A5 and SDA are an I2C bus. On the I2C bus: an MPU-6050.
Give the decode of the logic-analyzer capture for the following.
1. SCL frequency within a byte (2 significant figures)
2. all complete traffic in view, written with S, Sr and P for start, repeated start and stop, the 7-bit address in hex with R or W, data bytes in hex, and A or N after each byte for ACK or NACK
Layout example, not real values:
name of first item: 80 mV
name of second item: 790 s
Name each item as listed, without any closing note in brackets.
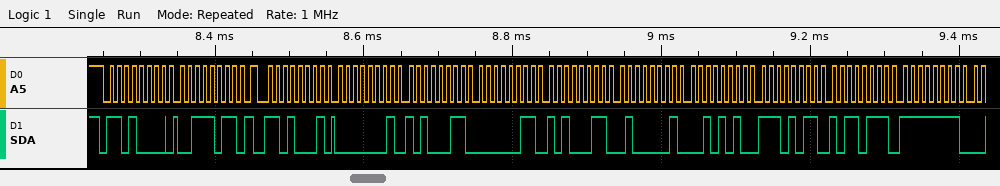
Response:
SCL frequency within a byte: 100 kHz
all complete traffic in view, written with S, Sr and P for start, repeated start and stop, the 7-bit address in hex with R or W, data bytes in hex, and A or N after each byte for ACK or NACK: S 68W A 3B A Sr 68R A 01 A A3 A 03 A A3 A 41 A 2A A EB A B7 A FF A
